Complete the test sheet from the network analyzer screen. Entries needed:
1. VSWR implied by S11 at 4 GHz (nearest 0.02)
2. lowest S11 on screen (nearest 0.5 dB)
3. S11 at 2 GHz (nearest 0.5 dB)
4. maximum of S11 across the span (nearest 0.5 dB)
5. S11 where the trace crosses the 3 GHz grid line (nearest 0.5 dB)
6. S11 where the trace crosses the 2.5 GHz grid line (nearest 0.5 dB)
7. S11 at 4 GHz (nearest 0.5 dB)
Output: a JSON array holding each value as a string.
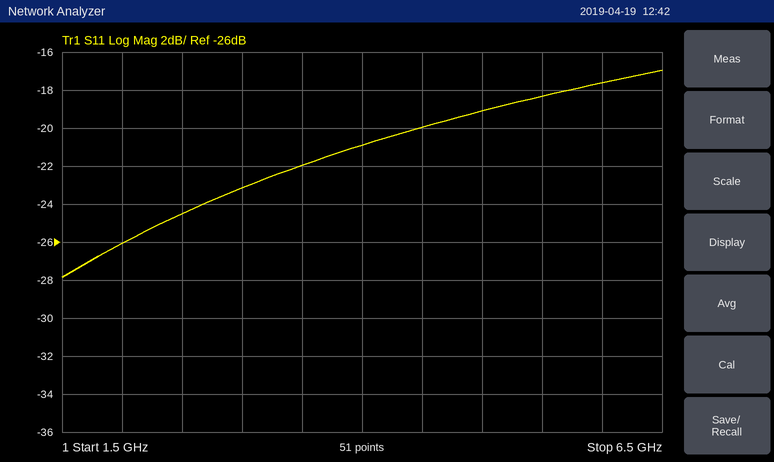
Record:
["1.20", "-28.0 dB", "-26.0 dB", "-17.0 dB", "-23.0 dB", "-24.5 dB", "-21.0 dB"]
